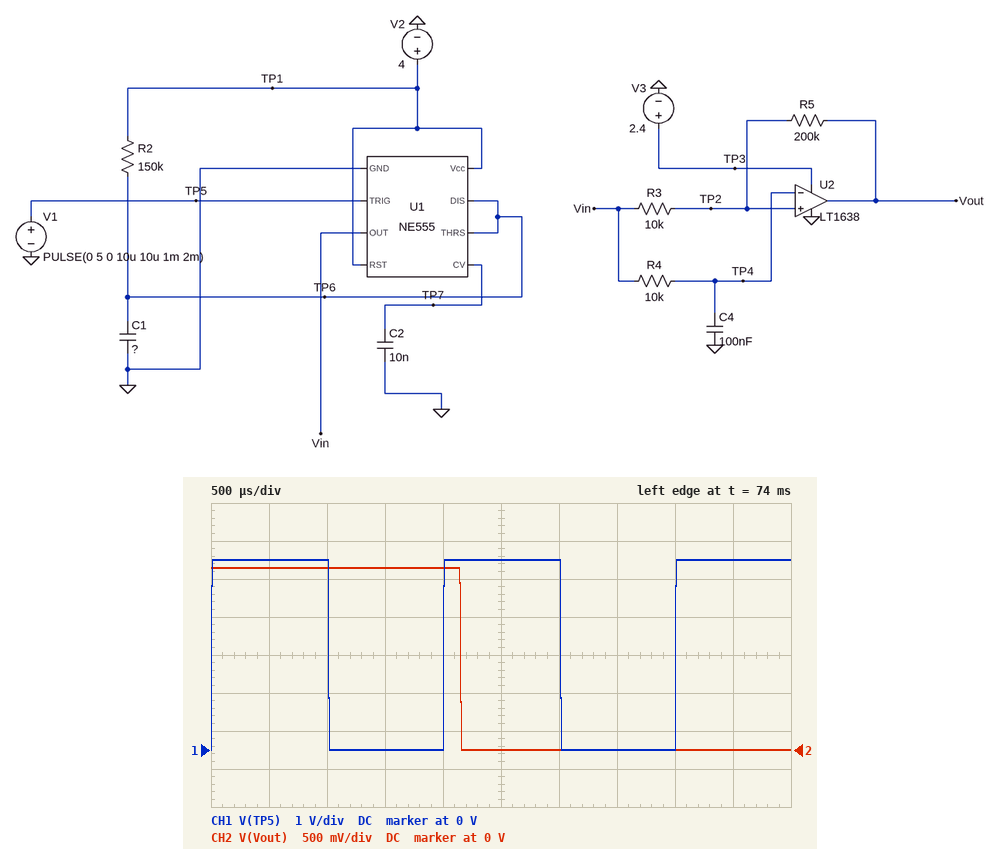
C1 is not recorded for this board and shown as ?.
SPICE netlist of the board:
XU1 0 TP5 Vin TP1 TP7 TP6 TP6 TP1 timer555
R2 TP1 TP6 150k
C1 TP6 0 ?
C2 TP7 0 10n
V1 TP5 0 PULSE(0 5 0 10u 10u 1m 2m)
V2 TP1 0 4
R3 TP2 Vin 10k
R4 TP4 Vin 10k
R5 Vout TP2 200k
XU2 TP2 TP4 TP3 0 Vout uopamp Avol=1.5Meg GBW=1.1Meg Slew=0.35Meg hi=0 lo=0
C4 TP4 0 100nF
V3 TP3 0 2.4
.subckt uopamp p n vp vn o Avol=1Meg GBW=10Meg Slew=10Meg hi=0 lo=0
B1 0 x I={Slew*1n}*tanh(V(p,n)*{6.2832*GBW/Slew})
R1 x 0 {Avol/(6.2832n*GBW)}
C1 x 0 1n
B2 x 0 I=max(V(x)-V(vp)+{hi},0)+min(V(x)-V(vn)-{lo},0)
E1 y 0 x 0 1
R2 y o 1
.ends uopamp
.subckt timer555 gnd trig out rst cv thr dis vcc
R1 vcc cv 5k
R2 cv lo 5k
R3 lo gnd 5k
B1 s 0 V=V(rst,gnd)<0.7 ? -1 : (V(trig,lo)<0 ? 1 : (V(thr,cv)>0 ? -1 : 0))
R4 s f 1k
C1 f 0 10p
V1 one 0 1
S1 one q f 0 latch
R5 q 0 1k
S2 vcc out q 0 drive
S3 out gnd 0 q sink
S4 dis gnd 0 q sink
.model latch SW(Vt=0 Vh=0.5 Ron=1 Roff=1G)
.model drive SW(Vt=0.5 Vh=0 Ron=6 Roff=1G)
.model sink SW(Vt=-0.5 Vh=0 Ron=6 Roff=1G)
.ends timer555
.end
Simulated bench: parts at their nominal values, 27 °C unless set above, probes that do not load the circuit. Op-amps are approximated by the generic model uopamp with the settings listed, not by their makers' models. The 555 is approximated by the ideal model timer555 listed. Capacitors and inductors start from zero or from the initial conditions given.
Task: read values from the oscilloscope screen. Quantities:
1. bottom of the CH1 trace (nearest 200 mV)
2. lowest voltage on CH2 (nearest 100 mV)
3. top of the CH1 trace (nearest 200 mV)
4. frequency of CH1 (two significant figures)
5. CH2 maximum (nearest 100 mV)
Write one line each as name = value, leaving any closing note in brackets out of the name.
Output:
bottom of the CH1 trace = 0 V
lowest voltage on CH2 = 0 V
top of the CH1 trace = 5.0 V
frequency of CH1 = 500 Hz
CH2 maximum = 2.4 V
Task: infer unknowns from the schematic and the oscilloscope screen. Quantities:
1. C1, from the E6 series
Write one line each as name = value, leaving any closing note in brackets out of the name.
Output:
C1, from the E6 series = 33 nF
